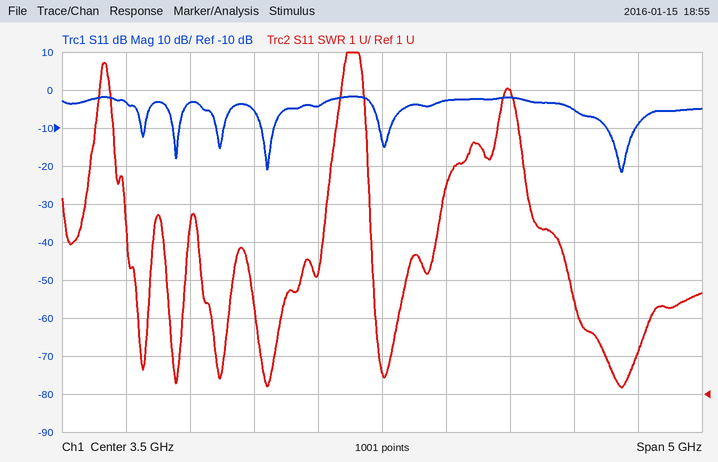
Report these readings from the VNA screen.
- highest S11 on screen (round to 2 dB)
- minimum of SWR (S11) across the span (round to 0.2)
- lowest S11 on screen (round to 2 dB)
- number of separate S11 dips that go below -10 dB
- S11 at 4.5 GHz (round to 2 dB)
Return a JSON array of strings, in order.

["-2 dB", "1.2", "-22 dB", "6", "-2 dB"]
